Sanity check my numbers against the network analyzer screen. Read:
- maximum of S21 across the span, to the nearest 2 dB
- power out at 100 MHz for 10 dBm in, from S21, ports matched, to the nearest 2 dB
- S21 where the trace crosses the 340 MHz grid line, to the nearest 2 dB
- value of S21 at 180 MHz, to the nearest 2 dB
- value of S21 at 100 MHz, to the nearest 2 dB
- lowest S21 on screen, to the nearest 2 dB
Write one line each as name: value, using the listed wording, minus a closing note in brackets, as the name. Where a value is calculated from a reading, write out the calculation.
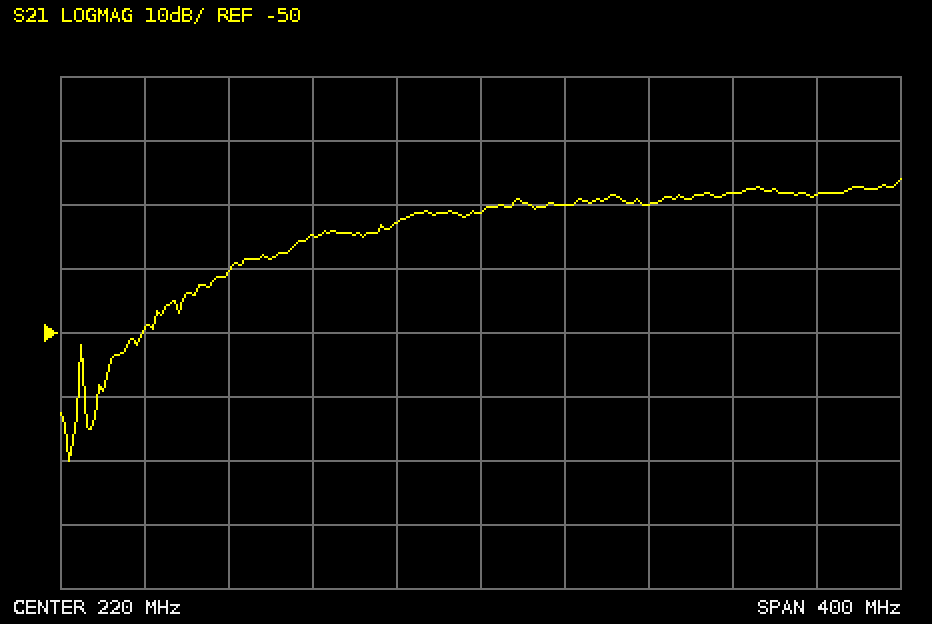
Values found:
maximum of S21 across the span, to the nearest 2 dB: -26 dB
power out at 100 MHz for 10 dBm in, from S21, ports matched, to the nearest 2 dB: 10 dBm + (-40 dB) = -30 dBm
S21 where the trace crosses the 340 MHz grid line, to the nearest 2 dB: -28 dB
value of S21 at 180 MHz, to the nearest 2 dB: -32 dB
value of S21 at 100 MHz, to the nearest 2 dB: -40 dB
lowest S21 on screen, to the nearest 2 dB: -70 dB
